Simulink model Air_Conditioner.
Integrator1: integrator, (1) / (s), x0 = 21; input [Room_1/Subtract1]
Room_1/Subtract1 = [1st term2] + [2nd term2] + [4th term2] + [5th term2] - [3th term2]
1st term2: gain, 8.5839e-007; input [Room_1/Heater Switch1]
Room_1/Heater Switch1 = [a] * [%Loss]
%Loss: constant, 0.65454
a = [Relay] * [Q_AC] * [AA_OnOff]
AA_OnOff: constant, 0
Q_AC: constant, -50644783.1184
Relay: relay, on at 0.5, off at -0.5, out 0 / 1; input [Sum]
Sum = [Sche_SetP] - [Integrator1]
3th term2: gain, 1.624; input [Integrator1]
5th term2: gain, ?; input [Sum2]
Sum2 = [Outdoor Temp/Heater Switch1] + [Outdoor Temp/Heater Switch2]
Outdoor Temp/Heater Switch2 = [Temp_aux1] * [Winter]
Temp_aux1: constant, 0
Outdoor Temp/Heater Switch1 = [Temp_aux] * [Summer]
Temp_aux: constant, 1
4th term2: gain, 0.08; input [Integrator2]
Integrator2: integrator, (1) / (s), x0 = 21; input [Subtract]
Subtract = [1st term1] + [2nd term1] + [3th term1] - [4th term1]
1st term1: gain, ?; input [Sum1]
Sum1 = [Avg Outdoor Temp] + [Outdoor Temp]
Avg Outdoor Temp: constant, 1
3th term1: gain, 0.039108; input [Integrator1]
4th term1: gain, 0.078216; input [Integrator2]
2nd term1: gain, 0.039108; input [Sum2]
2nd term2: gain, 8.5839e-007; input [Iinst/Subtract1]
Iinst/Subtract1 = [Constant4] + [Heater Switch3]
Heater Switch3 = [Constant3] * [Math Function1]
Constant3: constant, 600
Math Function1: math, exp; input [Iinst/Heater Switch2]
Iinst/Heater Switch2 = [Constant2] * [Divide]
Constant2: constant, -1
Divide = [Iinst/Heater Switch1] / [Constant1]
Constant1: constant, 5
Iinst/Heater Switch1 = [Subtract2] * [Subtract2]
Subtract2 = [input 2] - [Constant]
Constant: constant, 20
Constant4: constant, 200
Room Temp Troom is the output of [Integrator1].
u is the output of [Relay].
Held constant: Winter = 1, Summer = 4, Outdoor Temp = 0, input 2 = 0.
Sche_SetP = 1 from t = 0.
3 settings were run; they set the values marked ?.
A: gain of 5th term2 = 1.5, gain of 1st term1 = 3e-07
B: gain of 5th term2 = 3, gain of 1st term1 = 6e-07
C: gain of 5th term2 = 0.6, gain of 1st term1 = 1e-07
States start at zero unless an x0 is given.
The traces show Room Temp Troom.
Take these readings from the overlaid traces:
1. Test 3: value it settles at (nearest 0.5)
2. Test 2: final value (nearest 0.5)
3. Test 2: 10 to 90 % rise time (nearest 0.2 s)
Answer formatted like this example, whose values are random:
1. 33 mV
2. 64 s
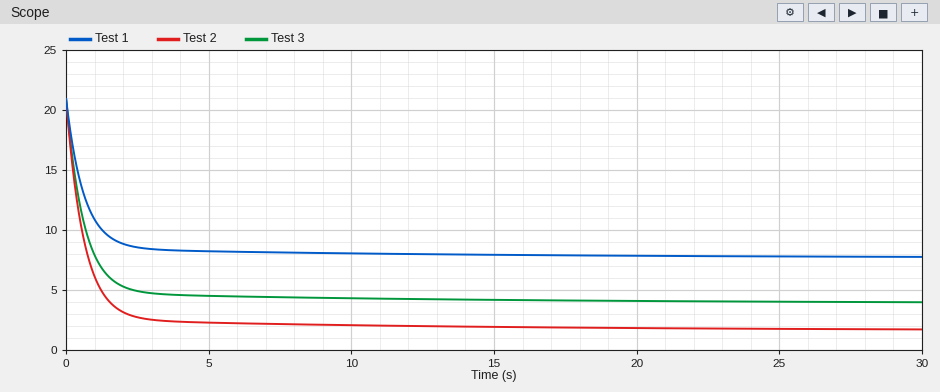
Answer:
1. 4.0
2. 1.5
3. 1.6 s
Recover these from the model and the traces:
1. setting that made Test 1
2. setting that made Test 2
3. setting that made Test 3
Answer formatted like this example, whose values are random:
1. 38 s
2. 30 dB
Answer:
1. B
2. C
3. A
